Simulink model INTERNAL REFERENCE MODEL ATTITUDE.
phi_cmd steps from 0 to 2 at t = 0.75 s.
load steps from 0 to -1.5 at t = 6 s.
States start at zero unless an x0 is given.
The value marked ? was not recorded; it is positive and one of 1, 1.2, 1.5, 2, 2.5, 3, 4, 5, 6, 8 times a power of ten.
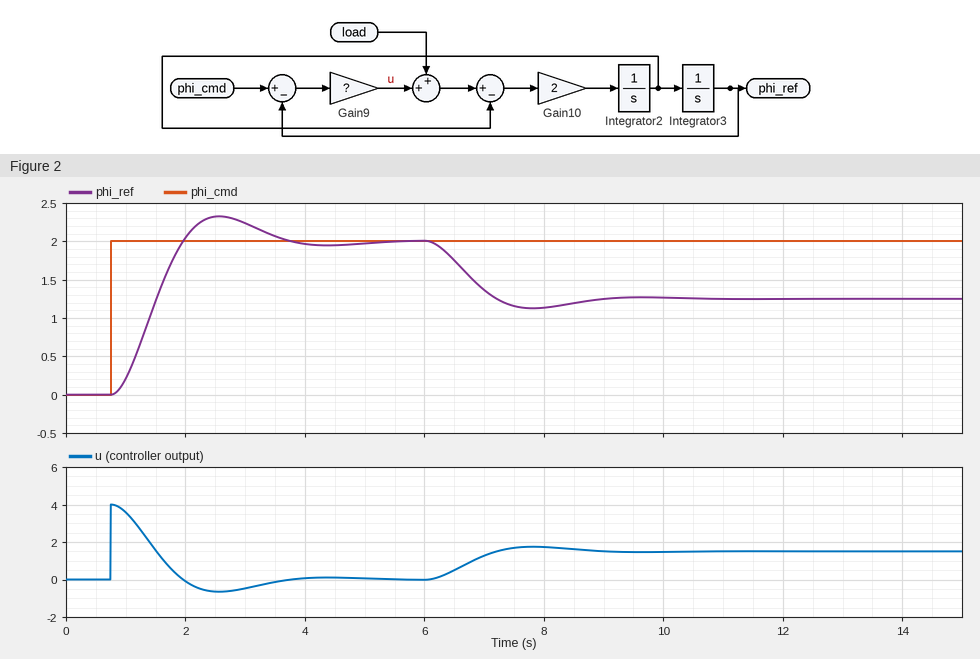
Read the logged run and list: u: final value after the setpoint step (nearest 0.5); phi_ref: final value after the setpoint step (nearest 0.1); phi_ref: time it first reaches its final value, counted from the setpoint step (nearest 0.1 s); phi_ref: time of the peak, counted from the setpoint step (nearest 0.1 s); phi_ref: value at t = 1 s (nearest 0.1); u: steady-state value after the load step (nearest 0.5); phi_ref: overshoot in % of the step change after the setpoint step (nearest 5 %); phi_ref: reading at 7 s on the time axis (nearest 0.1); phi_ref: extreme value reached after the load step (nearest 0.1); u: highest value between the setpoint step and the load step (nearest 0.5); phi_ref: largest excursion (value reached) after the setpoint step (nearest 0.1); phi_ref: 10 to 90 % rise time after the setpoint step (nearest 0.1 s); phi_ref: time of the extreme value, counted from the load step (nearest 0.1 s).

0.0
2.0
1.2 s
1.8 s
0.2
1.5
15 %
1.4
1.1
4.0
2.3
0.8 s
1.8 s
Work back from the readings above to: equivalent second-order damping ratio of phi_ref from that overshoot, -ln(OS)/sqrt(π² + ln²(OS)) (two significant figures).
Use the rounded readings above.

0.52
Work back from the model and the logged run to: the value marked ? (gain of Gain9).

2
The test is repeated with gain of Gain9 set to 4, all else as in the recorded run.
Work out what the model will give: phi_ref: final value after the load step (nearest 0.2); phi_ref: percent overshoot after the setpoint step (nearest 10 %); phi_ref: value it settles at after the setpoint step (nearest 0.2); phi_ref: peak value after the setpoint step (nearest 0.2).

1.6
30 %
2.0
2.6
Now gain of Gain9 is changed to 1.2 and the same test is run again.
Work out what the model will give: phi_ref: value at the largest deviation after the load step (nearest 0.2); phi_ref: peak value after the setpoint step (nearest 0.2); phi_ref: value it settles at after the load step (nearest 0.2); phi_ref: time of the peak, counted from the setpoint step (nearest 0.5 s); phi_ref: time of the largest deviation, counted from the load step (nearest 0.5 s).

0.6
2.2
0.8
2.5 s
2.5 s
